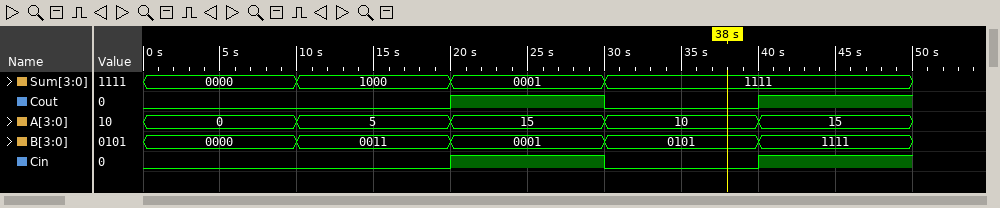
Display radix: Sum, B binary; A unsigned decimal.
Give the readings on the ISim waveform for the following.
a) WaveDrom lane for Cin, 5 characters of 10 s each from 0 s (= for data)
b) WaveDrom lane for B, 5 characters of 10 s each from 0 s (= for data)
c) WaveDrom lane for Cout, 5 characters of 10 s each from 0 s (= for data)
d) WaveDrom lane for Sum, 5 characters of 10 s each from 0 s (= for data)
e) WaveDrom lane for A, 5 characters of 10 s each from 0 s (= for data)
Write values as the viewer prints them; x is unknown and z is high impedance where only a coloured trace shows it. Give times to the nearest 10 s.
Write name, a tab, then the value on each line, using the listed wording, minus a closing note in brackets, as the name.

WaveDrom lane for Cin, 5 characters of 10 s each from 0 s	{name: 'Cin', wave: '0.101'}
WaveDrom lane for B, 5 characters of 10 s each from 0 s	{name: 'B', wave: '=====', data: '0000 0011 0001 0101 1111'}
WaveDrom lane for Cout, 5 characters of 10 s each from 0 s	{name: 'Cout', wave: '0.101'}
WaveDrom lane for Sum, 5 characters of 10 s each from 0 s	{name: 'Sum', wave: '====.', data: '0000 1000 0001 1111'}
WaveDrom lane for A, 5 characters of 10 s each from 0 s	{name: 'A', wave: '=====', data: '0 5 15 10 15'}
